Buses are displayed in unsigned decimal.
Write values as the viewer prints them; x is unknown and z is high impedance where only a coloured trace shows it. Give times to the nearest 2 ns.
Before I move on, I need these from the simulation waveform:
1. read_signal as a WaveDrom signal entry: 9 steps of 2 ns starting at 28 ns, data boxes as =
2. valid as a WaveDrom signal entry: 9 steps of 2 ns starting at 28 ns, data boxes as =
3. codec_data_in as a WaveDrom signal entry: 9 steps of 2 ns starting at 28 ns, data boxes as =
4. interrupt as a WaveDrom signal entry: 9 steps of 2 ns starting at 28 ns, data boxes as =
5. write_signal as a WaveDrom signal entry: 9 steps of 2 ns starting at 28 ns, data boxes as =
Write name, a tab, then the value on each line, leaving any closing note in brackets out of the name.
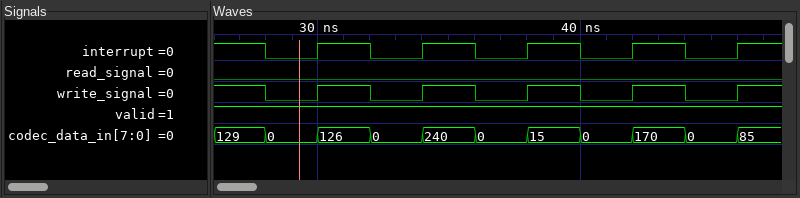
read_signal as a WaveDrom signal entry: 9 steps of 2 ns starting at 28 ns, data boxes as =	{name: 'read_signal', wave: '0........'}
valid as a WaveDrom signal entry: 9 steps of 2 ns starting at 28 ns, data boxes as =	{name: 'valid', wave: '1........'}
codec_data_in as a WaveDrom signal entry: 9 steps of 2 ns starting at 28 ns, data boxes as =	{name: 'codec_data_in', wave: '=========', data: '0 126 0 240 0 15 0 170 0'}
interrupt as a WaveDrom signal entry: 9 steps of 2 ns starting at 28 ns, data boxes as =	{name: 'interrupt', wave: '010101010'}
write_signal as a WaveDrom signal entry: 9 steps of 2 ns starting at 28 ns, data boxes as =	{name: 'write_signal', wave: '010101010'}
